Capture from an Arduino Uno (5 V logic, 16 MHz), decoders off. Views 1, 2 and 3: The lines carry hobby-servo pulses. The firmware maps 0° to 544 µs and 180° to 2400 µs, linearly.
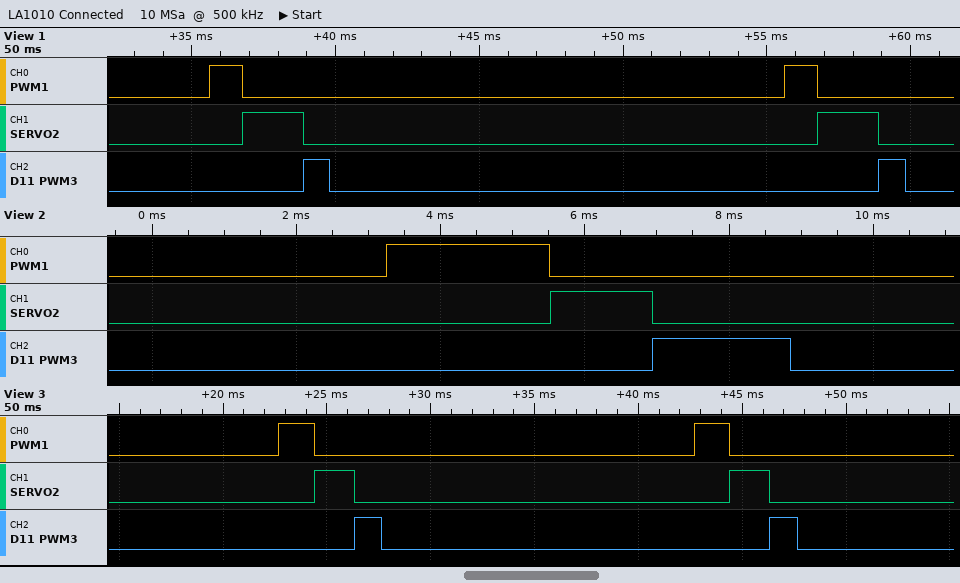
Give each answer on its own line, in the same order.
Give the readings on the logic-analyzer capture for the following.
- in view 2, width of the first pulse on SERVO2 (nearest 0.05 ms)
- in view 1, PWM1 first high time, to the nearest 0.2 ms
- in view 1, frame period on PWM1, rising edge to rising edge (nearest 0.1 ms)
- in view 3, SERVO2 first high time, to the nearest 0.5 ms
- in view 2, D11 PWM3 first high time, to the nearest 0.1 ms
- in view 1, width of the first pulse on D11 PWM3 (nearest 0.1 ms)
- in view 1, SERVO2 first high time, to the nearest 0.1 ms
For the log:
1.40 ms
1.2 ms
20.0 ms
2.0 ms
1.9 ms
0.9 ms
2.1 ms
